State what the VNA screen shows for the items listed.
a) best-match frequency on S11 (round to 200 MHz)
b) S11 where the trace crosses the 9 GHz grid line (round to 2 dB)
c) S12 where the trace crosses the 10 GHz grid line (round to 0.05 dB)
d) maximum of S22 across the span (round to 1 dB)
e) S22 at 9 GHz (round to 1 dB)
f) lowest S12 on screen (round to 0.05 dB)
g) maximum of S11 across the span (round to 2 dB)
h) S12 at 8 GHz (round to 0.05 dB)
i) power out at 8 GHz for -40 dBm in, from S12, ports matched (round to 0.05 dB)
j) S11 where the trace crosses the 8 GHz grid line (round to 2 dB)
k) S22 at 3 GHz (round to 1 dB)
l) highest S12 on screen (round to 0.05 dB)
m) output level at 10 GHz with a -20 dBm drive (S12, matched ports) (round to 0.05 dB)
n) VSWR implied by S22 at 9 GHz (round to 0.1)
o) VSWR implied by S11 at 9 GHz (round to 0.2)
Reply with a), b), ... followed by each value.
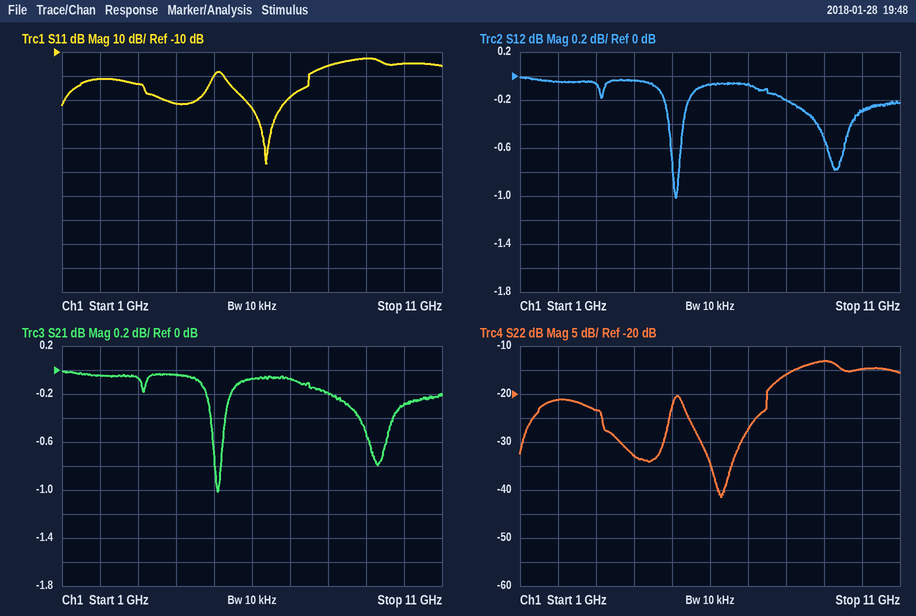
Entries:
a) 6.4 GHz
b) -12 dB
c) -0.30 dB
d) -13 dB
e) -13 dB
f) -1.00 dB
g) -12 dB
h) -0.20 dB
i) -40.20 dBm
j) -16 dB
k) -23 dB
l) 0.00 dB
m) -20.30 dBm
n) 1.6
o) 1.6
